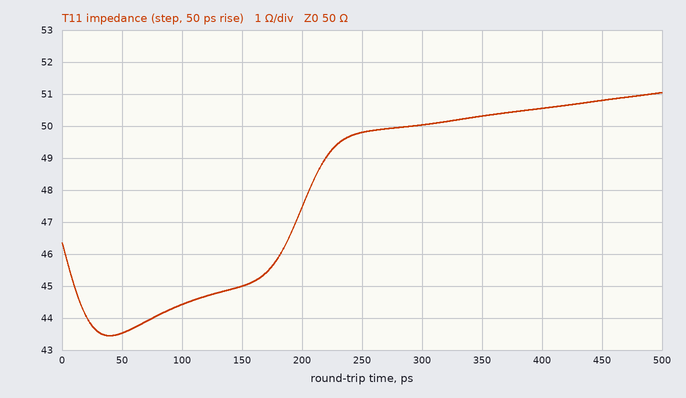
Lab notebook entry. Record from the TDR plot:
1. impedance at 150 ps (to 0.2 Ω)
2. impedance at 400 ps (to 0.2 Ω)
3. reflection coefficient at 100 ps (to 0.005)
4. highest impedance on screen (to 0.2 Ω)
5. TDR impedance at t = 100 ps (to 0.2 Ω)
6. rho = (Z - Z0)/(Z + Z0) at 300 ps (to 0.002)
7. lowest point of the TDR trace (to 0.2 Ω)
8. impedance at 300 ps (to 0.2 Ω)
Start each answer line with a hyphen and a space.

- 45.0 Ω
- 50.6 Ω
- -0.060
- 51.0 Ω
- 44.4 Ω
- 0.000
- 43.4 Ω
- 50.0 Ω
